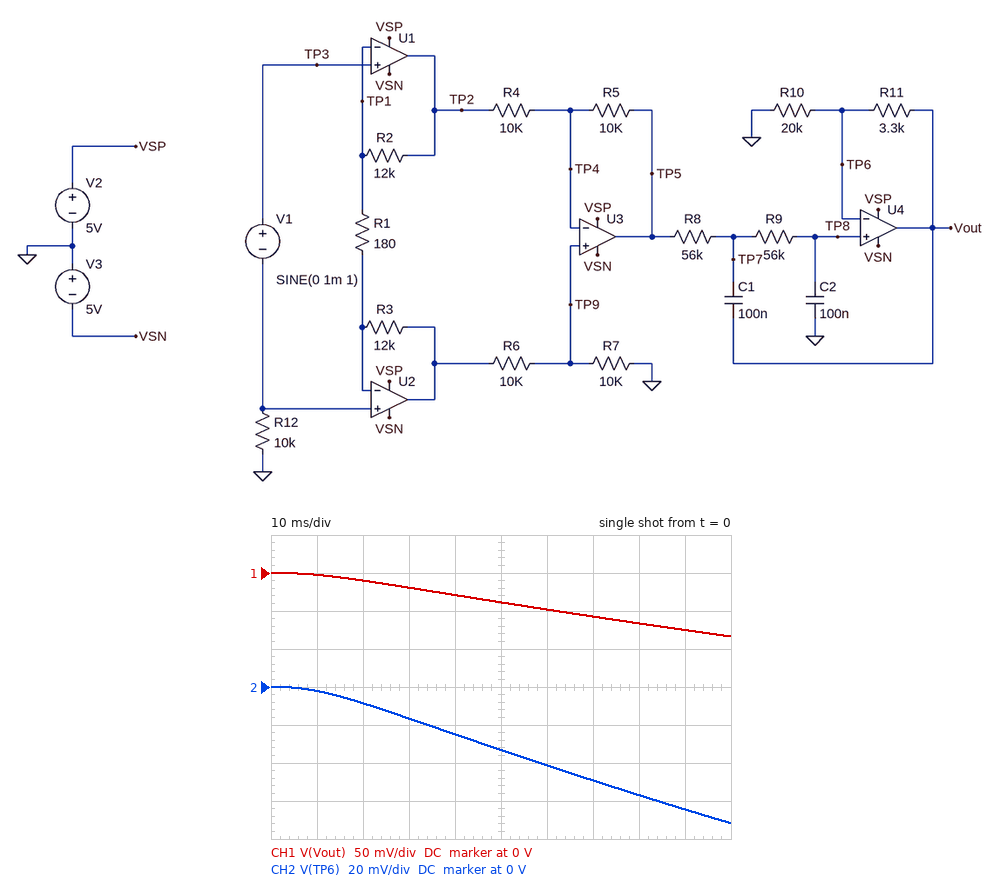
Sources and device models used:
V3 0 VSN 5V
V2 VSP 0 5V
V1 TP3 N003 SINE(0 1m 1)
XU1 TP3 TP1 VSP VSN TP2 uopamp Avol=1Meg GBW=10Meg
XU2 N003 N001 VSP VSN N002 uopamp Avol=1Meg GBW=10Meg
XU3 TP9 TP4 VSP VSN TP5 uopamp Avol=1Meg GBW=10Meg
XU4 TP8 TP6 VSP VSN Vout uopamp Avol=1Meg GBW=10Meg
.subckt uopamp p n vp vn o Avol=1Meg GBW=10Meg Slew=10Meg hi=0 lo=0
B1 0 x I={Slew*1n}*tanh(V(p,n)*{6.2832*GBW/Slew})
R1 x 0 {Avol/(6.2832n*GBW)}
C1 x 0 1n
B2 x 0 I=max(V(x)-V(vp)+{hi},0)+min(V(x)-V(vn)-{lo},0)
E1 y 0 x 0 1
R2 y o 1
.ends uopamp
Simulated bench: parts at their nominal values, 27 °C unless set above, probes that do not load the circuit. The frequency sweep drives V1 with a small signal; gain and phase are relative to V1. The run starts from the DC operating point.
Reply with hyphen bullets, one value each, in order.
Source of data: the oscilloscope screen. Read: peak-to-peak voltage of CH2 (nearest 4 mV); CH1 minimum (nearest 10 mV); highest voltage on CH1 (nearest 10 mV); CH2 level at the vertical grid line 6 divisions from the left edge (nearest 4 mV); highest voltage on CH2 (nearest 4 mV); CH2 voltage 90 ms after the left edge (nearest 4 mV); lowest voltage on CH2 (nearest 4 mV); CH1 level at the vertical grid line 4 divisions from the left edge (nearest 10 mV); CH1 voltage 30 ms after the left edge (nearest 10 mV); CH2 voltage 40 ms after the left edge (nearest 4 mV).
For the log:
- 72 mV
- -80 mV
- 0 V
- -40 mV
- 0 V
- -64 mV
- -72 mV
- -30 mV
- -20 mV
- -24 mV
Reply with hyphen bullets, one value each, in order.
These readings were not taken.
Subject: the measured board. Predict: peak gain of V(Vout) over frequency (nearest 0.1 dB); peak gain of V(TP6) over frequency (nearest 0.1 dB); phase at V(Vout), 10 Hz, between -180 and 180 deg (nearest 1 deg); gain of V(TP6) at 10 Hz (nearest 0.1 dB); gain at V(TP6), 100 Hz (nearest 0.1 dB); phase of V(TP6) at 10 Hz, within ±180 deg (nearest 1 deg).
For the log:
- 43.9 dB
- 42.6 dB
- 144 deg
- 41.8 dB
- 20.2 dB
- 144 deg
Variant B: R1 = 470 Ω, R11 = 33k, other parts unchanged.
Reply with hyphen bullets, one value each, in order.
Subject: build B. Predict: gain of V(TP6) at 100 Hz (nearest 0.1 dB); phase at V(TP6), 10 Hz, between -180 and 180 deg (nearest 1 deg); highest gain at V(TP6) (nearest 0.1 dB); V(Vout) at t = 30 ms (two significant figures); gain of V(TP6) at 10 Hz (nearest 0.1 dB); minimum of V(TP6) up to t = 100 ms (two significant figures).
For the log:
- 13.2 dB
- 172 deg
- 43.6 dB
- -26 mV
- 35.4 dB
- -30 mV
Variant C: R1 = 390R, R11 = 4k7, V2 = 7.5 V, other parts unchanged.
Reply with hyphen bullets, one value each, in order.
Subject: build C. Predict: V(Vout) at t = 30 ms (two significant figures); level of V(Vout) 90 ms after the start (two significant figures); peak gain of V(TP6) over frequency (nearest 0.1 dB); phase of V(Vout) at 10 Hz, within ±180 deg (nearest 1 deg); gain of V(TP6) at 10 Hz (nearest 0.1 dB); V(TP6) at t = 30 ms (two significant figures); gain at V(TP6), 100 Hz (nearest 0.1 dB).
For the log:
- -9.7 mV
- -37 mV
- 35.9 dB
- 145 deg
- 35.3 dB
- -7.9 mV
- 13.7 dB
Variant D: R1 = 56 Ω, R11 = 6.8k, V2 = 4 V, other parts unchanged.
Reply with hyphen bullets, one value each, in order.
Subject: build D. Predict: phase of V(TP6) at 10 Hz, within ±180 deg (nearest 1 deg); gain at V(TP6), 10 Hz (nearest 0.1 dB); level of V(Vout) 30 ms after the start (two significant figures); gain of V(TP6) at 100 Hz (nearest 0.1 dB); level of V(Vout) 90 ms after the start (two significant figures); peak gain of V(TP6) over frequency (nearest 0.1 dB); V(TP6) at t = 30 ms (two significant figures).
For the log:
- 146 deg
- 52.2 dB
- -74 mV
- 30.5 dB
- -280 mV
- 52.7 dB
- -55 mV
